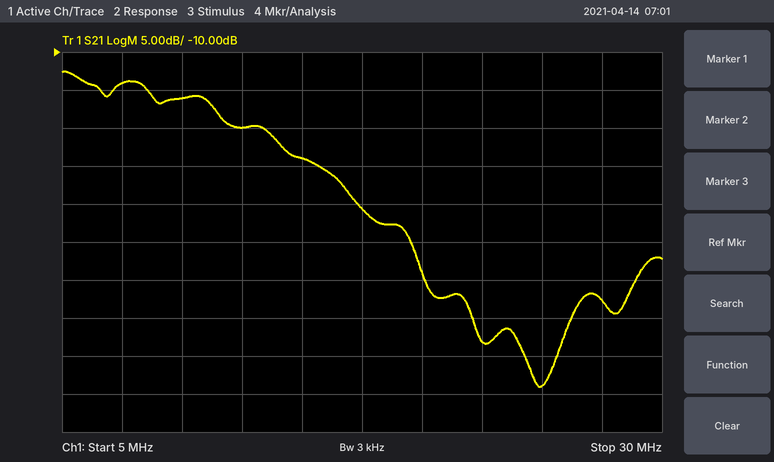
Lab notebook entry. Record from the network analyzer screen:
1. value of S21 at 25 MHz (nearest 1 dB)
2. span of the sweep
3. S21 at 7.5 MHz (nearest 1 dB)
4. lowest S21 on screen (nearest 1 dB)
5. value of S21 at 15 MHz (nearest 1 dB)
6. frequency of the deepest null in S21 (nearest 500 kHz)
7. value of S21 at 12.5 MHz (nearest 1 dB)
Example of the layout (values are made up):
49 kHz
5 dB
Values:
-54 dB
25 MHz
-14 dB
-54 dB
-24 dB
25.0 MHz
-20 dB
